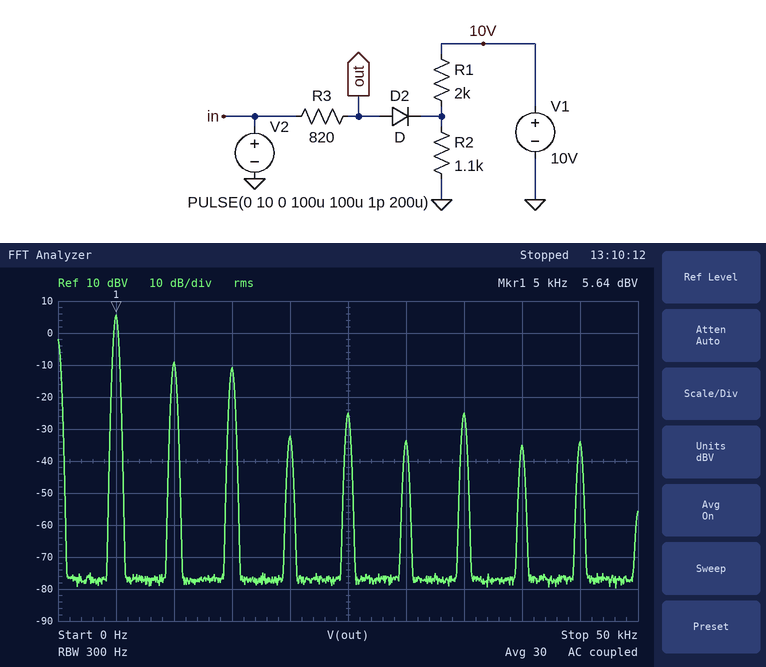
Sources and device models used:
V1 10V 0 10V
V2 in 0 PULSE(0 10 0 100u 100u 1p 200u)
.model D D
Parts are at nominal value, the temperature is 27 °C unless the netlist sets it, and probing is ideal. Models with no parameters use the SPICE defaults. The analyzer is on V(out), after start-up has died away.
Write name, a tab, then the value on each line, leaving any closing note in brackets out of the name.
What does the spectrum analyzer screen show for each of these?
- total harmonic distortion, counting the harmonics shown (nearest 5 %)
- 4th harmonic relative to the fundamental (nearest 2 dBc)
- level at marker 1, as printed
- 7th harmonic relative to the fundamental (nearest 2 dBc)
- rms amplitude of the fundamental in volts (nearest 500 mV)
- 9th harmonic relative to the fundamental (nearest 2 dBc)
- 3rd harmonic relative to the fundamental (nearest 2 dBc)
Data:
total harmonic distortion, counting the harmonics shown	25 %
4th harmonic relative to the fundamental	-38 dBc
level at marker 1, as printed	5.64 dBV
7th harmonic relative to the fundamental	-30 dBc
rms amplitude of the fundamental in volts	2.0 V
9th harmonic relative to the fundamental	-40 dBc
3rd harmonic relative to the fundamental	-16 dBc
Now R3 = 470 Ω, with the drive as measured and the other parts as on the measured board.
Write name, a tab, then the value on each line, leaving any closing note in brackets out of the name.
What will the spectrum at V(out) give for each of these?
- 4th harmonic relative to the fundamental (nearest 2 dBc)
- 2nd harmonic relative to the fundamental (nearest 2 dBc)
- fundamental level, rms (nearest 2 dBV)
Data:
4th harmonic relative to the fundamental	-42 dBc
2nd harmonic relative to the fundamental	-18 dBc
fundamental level, rms	6 dBV
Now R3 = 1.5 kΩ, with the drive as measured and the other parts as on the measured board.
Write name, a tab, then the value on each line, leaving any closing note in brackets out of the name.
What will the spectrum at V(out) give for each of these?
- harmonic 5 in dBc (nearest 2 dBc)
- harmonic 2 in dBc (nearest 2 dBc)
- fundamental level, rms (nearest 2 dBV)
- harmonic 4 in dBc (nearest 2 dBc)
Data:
harmonic 5 in dBc	-32 dBc
harmonic 2 in dBc	-12 dBc
fundamental level, rms	4 dBV
harmonic 4 in dBc	-34 dBc
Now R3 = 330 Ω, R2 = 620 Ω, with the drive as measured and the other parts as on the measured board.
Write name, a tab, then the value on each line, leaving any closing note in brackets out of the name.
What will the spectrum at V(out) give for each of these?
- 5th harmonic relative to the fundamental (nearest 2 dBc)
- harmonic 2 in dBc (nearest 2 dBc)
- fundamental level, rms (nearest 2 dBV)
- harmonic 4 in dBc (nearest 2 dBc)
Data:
5th harmonic relative to the fundamental	-26 dBc
harmonic 2 in dBc	-20 dBc
fundamental level, rms	6 dBV
harmonic 4 in dBc	-30 dBc
